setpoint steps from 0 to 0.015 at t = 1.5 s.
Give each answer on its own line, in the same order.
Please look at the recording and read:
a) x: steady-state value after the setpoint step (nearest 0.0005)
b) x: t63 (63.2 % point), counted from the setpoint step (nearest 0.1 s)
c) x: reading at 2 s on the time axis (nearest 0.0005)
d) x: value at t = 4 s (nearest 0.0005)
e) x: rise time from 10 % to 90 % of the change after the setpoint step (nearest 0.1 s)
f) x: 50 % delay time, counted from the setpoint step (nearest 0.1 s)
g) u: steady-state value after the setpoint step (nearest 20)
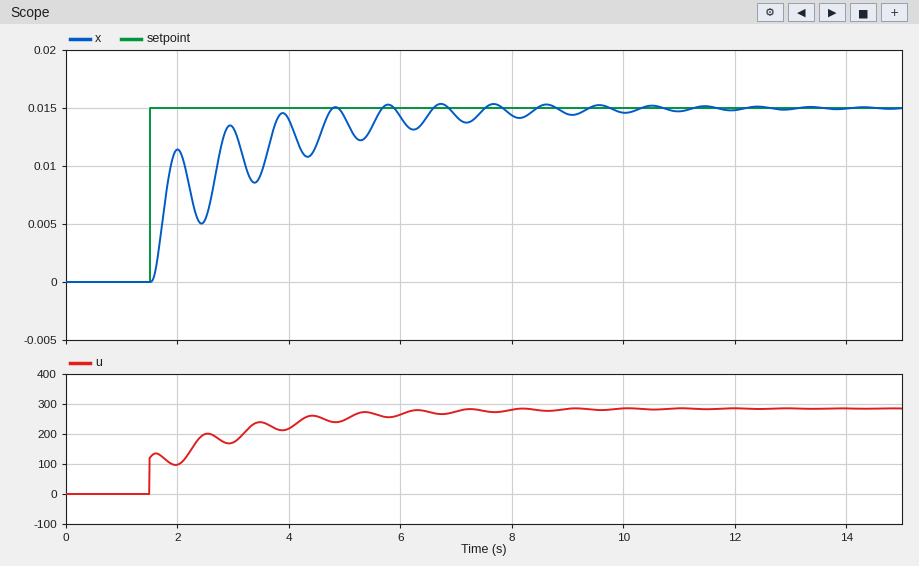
0.0150
0.4 s
0.0115
0.0140
2.1 s
0.3 s
280
